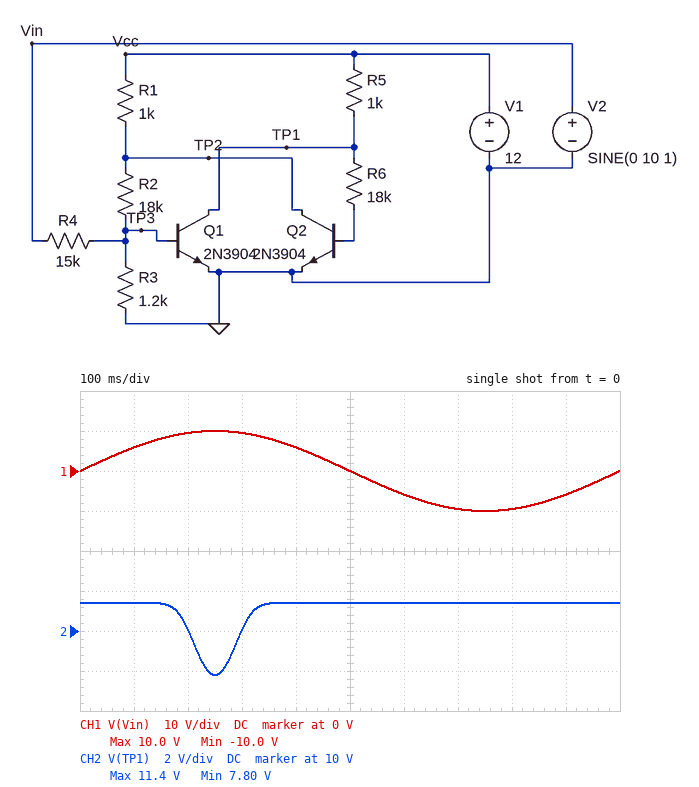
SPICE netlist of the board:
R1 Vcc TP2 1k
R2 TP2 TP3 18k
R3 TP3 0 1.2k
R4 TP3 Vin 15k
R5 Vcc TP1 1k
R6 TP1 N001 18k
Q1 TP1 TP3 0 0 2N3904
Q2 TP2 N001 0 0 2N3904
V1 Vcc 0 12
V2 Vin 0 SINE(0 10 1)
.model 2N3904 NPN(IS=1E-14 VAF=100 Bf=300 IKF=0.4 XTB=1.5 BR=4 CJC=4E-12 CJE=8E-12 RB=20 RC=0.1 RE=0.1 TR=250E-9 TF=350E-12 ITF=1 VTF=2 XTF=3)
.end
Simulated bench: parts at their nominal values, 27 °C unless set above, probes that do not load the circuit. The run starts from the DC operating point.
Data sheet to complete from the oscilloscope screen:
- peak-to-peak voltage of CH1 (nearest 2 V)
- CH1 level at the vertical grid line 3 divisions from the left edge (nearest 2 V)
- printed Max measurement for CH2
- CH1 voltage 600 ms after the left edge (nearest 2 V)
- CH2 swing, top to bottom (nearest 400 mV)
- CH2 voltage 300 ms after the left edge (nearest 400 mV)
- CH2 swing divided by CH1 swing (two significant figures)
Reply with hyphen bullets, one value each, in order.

- 20 V
- 10 V
- 11.4 V
- -6 V
- 3.6 V
- 10.0 V
- 0.18
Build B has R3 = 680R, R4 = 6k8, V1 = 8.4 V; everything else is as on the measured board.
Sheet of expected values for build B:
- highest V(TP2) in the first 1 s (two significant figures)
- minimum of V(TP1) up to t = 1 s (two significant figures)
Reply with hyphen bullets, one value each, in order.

- 8.0 V
- 41 mV
